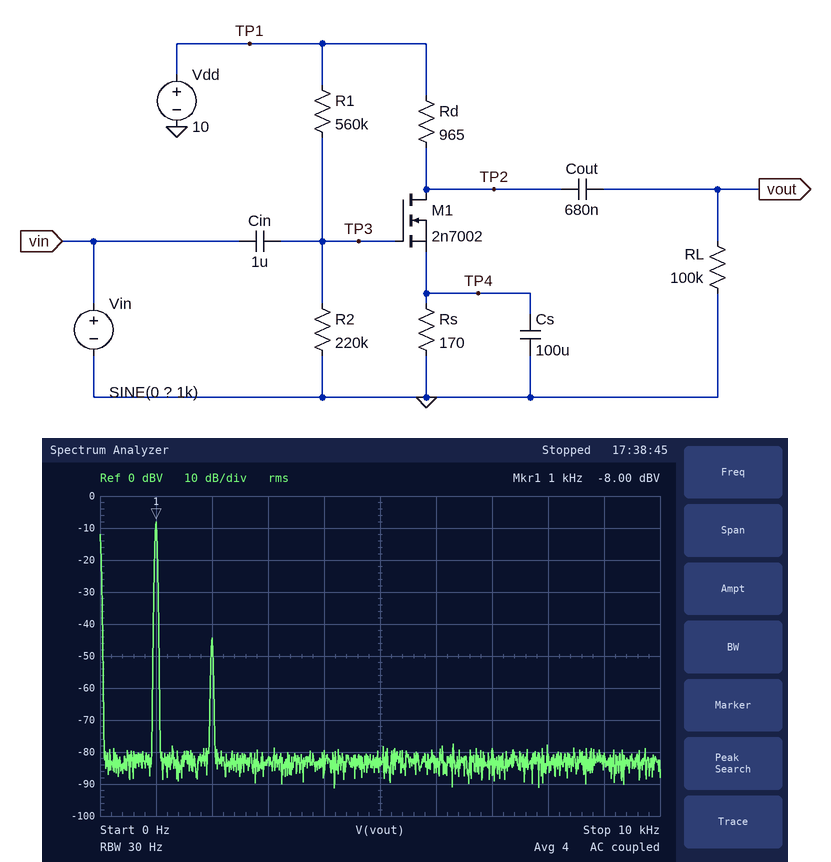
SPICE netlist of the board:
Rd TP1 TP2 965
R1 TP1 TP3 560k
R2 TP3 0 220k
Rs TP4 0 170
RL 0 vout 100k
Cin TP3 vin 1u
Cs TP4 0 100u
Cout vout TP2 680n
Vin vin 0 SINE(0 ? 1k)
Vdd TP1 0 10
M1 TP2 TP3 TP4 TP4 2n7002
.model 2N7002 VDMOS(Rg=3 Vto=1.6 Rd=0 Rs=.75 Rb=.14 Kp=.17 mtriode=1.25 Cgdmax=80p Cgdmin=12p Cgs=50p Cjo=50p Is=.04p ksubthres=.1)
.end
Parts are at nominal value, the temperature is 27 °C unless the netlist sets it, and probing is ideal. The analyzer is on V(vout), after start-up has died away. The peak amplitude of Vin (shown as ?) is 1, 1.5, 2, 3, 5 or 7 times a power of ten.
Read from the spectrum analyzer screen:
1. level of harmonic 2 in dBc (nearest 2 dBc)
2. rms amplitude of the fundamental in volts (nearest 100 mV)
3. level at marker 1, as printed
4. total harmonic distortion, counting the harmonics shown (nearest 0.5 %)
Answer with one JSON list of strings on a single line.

["-36 dBc", "400 mV", "-8.00 dBV", "1.5 %"]
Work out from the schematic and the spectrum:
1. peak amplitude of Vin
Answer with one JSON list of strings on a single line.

["15 mV"]
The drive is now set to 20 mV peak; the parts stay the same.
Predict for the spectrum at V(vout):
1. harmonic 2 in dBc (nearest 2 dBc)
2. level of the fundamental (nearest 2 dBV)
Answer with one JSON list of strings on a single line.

["-34 dBc", "-6 dBV"]
